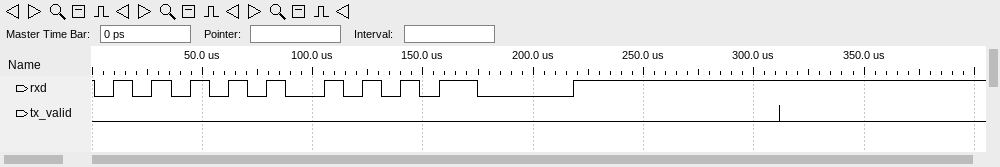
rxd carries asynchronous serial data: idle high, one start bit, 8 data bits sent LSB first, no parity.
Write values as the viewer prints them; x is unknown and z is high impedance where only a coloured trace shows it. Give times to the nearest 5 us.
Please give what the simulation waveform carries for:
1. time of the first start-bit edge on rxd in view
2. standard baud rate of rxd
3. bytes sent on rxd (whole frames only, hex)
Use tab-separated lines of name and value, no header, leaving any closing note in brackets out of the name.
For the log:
time of the first start-bit edge on rxd in view	0 us
standard baud rate of rxd	115200 baud
bytes sent on rxd	55, AA, F0
